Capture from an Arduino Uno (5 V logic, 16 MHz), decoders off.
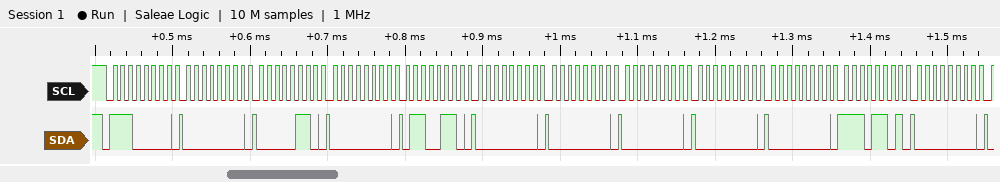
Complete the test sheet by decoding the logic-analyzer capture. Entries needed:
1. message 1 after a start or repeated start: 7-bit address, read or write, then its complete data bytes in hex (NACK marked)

0x70 write: 00 06 00 66 00 00 00 00 00 ED 00
